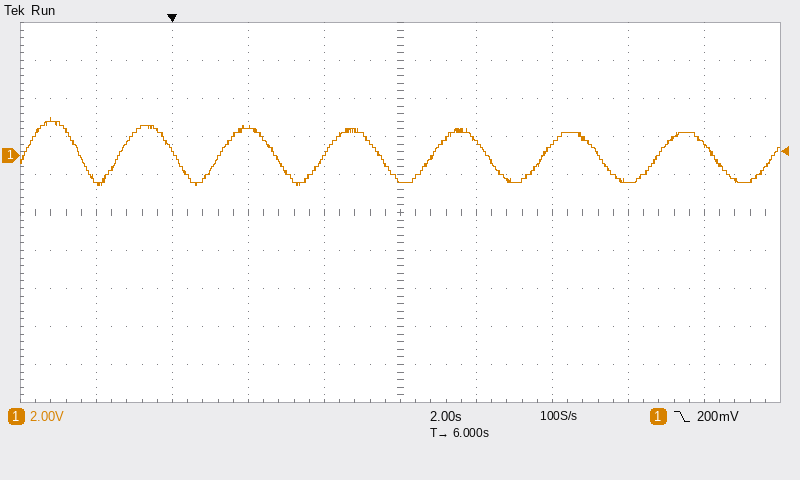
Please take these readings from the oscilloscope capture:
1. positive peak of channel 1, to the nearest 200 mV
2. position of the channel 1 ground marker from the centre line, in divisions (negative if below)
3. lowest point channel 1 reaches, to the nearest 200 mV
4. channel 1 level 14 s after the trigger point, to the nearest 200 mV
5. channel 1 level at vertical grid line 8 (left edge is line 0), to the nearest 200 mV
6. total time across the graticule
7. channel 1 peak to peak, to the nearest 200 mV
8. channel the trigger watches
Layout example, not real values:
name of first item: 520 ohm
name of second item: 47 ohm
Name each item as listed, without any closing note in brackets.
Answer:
positive peak of channel 1, to the nearest 200 mV: 2.0 V
position of the channel 1 ground marker from the centre line, in divisions: +1.5 div
lowest point channel 1 reaches, to the nearest 200 mV: -1.6 V
channel 1 level 14 s after the trigger point, to the nearest 200 mV: 600 mV
channel 1 level at vertical grid line 8 (left edge is line 0), to the nearest 200 mV: -1.4 V
total time across the graticule: 20 s
channel 1 peak to peak, to the nearest 200 mV: 3.6 V
channel the trigger watches: channel 1
